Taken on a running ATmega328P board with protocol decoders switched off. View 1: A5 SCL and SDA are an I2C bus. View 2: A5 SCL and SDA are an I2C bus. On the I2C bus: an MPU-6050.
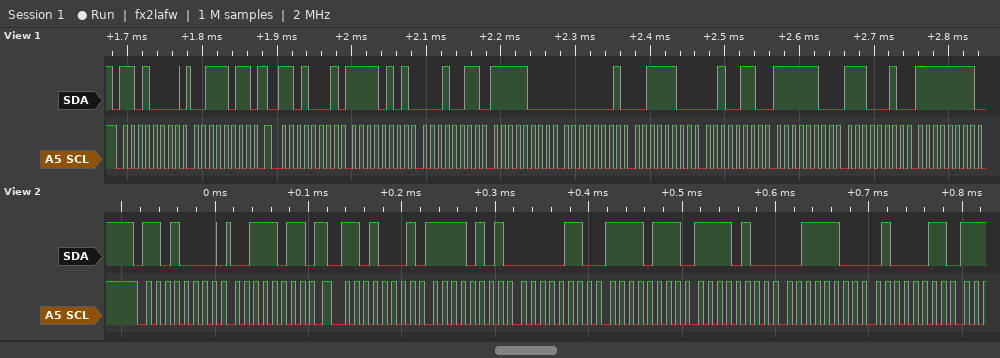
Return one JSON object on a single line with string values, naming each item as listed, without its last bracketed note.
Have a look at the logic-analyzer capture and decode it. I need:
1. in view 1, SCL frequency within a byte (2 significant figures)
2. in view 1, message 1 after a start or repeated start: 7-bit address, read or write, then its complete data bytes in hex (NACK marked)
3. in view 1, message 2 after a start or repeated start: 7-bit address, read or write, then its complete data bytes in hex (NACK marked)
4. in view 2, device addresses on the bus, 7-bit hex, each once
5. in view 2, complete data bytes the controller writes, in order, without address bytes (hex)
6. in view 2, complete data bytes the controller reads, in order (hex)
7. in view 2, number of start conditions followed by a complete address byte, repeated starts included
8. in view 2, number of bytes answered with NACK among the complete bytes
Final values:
{"in view 1, SCL frequency within a byte": "100 kHz", "in view 1, message 1 after a start or repeated start: 7-bit address, read or write, then its complete data bytes in hex": "0x68 write: 3B", "in view 1, message 2 after a start or repeated start: 7-bit address, read or write, then its complete data bytes in hex": "0x68 read: F5 13 F8 01 3C 26 FC E2 FF", "in view 2, device addresses on the bus, 7-bit hex, each once": "0x68", "in view 2, complete data bytes the controller writes, in order, without address bytes": "3B", "in view 2, complete data bytes the controller reads, in order": "F5 06 F7 F4 3C 43", "in view 2, number of start conditions followed by a complete address byte, repeated starts included": "2", "in view 2, number of bytes answered with NACK among the complete bytes": "0"}
